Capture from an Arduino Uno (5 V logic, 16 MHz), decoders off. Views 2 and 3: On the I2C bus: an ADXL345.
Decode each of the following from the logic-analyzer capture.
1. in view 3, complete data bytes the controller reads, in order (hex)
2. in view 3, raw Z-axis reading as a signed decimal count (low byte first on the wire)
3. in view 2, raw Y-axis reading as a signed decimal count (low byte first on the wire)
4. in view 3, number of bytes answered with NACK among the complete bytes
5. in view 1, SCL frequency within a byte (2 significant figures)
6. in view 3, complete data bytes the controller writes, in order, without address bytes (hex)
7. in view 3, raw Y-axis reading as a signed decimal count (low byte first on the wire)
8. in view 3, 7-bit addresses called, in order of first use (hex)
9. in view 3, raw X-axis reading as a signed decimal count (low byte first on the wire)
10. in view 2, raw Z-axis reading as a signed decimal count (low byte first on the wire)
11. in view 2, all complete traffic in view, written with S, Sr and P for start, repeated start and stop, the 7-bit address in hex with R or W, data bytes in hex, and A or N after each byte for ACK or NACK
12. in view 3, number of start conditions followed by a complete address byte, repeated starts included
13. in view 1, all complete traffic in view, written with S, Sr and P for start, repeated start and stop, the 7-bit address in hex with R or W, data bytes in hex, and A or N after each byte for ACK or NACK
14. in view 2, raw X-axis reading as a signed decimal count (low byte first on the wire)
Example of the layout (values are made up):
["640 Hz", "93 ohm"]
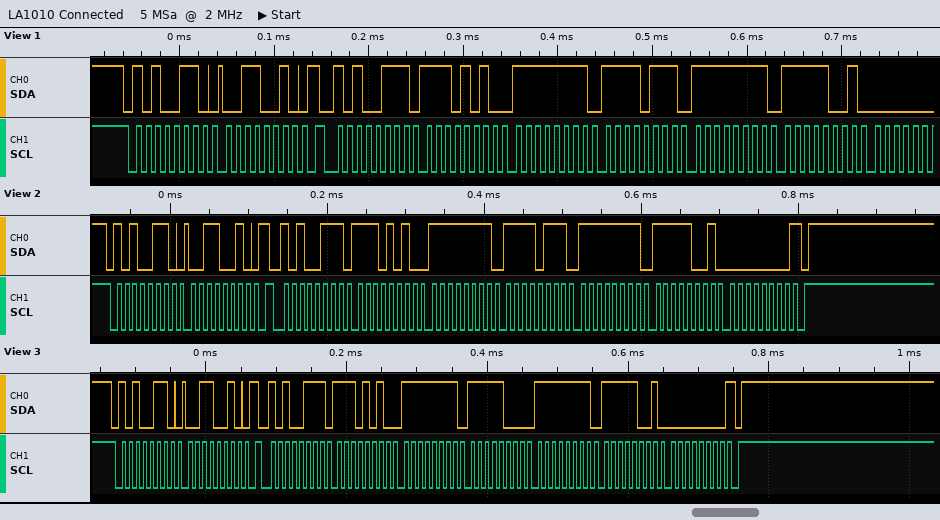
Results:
["EA FF F8 FF F9 00", "249", "-9", "1", "100 kHz", "32", "-8", "0x53", "-22", "249", "S 53W A 32 A Sr 53R A EA A FF A F7 A FF A F9 A 00 N P", "2", "S 53W A 32 A Sr 53R A EA A FF A F7 A FF A F9 A", "-22"]
